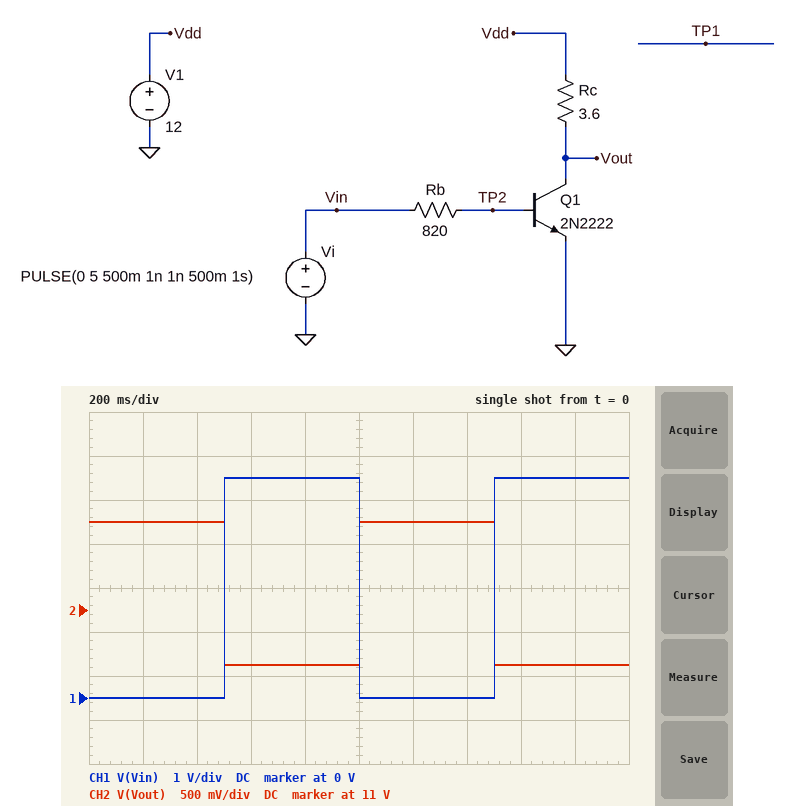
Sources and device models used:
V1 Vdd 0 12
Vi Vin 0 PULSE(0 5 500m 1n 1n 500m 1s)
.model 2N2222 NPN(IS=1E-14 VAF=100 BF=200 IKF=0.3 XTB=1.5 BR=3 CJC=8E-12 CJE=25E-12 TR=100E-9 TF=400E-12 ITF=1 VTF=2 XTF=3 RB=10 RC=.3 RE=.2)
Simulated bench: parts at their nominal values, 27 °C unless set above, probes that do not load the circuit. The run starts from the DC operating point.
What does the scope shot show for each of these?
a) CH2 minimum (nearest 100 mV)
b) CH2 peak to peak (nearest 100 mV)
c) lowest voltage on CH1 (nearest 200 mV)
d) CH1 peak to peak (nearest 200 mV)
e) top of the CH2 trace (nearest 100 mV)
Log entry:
10.4 V
1.6 V
0 V
5.0 V
12.0 V
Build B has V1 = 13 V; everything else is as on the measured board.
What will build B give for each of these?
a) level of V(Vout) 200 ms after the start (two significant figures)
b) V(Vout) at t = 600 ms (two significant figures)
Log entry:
13 V
11 V
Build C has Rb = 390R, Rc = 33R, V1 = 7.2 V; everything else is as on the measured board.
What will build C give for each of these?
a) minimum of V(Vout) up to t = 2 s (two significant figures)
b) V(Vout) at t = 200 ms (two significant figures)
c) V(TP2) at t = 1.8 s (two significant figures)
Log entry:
180 mV
7.2 V
960 mV
